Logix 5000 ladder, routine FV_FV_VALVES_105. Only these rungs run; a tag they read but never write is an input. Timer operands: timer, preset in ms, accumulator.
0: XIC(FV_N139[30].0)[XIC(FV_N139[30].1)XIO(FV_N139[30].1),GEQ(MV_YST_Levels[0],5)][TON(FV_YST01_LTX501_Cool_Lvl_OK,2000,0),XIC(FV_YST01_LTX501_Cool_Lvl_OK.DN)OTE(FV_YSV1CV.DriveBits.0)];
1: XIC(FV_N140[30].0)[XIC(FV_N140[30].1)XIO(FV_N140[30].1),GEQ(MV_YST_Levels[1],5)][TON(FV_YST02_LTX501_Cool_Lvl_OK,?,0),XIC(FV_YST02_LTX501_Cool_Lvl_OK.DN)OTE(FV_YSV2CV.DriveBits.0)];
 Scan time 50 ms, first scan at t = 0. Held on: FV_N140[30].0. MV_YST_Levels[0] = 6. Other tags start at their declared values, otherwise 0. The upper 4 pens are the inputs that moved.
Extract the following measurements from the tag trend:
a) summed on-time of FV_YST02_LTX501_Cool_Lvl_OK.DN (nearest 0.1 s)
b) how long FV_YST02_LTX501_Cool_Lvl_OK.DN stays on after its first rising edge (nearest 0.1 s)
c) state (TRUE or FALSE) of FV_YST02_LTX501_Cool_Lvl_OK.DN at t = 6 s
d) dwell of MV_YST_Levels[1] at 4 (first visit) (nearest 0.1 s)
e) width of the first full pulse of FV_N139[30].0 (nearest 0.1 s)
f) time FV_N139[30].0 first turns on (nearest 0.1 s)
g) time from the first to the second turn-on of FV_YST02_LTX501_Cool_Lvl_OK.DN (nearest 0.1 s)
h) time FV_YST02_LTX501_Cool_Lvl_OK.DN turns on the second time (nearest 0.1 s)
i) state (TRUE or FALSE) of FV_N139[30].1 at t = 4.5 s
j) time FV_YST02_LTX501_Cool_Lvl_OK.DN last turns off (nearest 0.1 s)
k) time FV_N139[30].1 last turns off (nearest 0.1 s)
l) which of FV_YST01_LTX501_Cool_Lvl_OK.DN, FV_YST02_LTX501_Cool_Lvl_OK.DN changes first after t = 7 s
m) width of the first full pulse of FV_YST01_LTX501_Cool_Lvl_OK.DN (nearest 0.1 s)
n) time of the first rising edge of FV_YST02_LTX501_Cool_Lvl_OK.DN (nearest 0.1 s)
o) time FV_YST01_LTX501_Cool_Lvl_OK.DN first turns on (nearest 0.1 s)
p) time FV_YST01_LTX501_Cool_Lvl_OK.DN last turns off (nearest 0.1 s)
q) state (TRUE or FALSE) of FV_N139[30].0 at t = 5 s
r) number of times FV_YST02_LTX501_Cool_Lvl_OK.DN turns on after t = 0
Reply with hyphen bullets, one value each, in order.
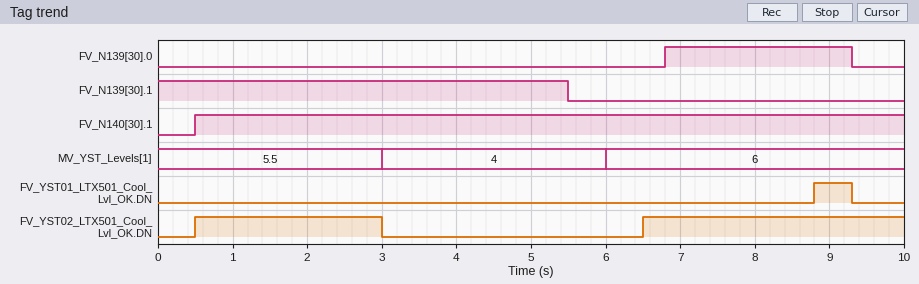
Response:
- 6.0 s
- 2.5 s
- FALSE
- 3.0 s
- 2.5 s
- 6.8 s
- 6.0 s
- 6.5 s
- TRUE
- 3.0 s
- 5.5 s
- FV_YST01_LTX501_Cool_Lvl_OK.DN
- 0.5 s
- 0.5 s
- 8.8 s
- 9.3 s
- FALSE
- 2
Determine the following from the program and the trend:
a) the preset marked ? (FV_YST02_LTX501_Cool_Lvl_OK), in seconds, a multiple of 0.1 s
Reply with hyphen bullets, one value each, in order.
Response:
- 0.5 s
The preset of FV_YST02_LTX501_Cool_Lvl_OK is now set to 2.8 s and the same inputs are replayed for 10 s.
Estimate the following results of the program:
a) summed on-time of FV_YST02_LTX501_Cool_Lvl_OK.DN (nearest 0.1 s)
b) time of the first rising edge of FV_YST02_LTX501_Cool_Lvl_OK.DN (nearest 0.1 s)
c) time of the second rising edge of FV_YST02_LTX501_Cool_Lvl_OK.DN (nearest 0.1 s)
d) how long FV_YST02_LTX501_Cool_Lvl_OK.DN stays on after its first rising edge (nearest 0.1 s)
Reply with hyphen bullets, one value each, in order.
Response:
- 1.4 s
- 2.8 s
- 8.8 s
- 0.2 s
